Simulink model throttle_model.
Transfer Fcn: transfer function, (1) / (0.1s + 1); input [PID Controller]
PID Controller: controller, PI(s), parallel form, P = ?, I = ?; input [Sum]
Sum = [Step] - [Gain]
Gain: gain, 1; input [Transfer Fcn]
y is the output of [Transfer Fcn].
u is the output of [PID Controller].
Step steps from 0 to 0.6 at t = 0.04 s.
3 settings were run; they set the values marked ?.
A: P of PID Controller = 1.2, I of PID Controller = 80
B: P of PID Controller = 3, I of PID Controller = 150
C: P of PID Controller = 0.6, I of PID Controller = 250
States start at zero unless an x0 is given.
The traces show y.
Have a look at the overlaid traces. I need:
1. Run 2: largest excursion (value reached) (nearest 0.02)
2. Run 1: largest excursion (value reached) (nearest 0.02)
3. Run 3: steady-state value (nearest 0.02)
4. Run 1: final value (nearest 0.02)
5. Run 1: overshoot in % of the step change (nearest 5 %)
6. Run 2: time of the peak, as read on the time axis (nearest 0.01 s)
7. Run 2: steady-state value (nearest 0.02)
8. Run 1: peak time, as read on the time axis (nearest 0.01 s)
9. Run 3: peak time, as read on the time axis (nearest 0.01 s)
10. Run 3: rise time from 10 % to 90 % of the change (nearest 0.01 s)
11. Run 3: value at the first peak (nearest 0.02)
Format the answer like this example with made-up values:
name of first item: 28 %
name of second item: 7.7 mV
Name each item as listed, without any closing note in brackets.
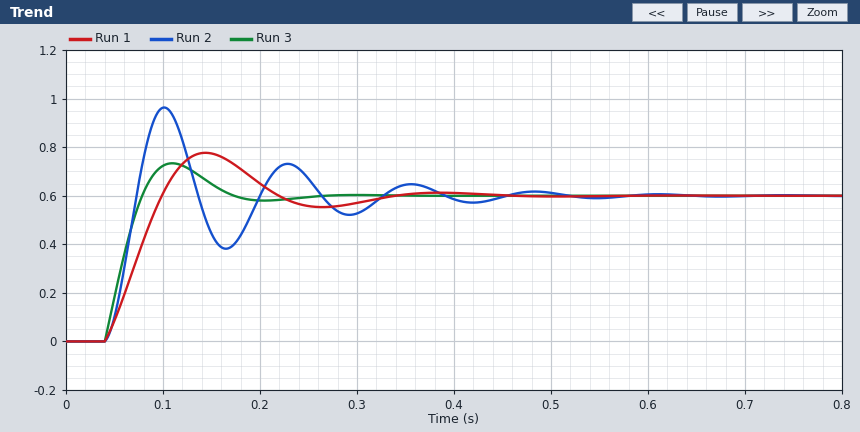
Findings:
Run 2: largest excursion (value reached): 0.96
Run 1: largest excursion (value reached): 0.78
Run 3: steady-state value: 0.60
Run 1: final value: 0.60
Run 1: overshoot in % of the step change: 30 %
Run 2: time of the peak, as read on the time axis: 0.10 s
Run 2: steady-state value: 0.60
Run 1: peak time, as read on the time axis: 0.14 s
Run 3: peak time, as read on the time axis: 0.11 s
Run 3: rise time from 10 % to 90 % of the change: 0.03 s
Run 3: value at the first peak: 0.74
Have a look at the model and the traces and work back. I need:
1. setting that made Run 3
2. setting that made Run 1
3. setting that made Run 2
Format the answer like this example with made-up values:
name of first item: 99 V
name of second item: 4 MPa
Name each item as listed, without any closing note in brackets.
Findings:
setting that made Run 3: B
setting that made Run 1: A
setting that made Run 2: C
